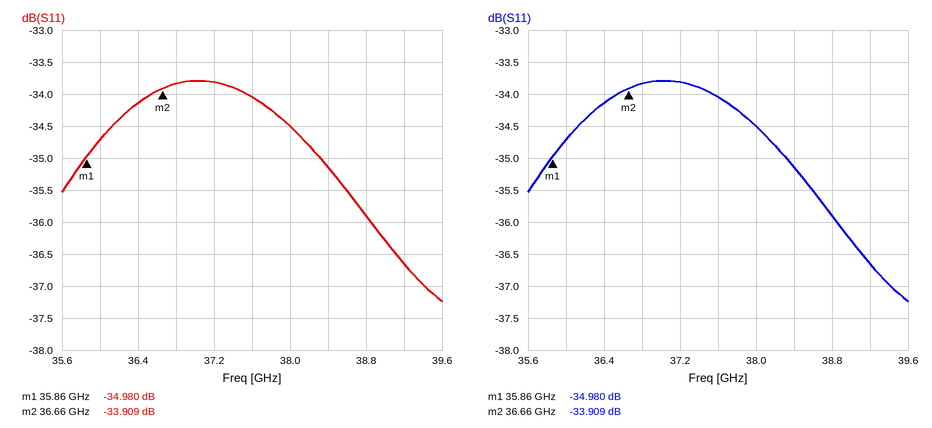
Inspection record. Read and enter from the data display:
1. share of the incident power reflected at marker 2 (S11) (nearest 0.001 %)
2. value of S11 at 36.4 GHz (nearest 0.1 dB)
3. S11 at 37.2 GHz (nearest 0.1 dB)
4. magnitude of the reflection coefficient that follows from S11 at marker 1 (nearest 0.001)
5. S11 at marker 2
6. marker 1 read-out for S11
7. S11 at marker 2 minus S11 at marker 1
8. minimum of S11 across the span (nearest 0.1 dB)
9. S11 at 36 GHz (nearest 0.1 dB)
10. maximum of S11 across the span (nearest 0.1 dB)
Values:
0.041 %
-34.1 dB
-33.8 dB
0.018
-33.909 dB
-34.980 dB
1.071 dB
-37.2 dB
-34.7 dB
-33.8 dB
